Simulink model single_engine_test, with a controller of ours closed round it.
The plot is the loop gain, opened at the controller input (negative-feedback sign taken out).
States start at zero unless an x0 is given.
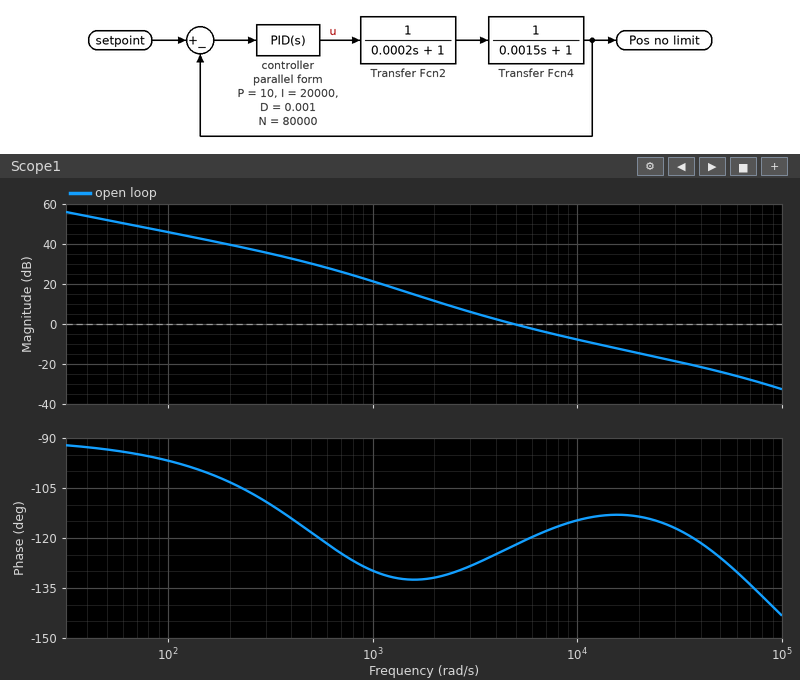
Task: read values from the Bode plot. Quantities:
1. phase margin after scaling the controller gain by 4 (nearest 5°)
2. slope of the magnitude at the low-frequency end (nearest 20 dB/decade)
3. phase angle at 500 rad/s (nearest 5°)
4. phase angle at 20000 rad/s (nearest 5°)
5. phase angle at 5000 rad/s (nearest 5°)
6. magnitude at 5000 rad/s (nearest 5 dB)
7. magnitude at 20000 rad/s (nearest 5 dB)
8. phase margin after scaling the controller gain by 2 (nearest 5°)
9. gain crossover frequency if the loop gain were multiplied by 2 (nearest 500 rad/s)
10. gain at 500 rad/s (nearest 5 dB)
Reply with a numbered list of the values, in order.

1. 65°
2. -20 dB/decade
3. -120°
4. -115°
5. -120°
6. 0 dB
7. -15 dB
8. 65°
9. 8500 rad/s
10. 30 dB
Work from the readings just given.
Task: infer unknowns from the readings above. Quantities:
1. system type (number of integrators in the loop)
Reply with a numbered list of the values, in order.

1. 1
